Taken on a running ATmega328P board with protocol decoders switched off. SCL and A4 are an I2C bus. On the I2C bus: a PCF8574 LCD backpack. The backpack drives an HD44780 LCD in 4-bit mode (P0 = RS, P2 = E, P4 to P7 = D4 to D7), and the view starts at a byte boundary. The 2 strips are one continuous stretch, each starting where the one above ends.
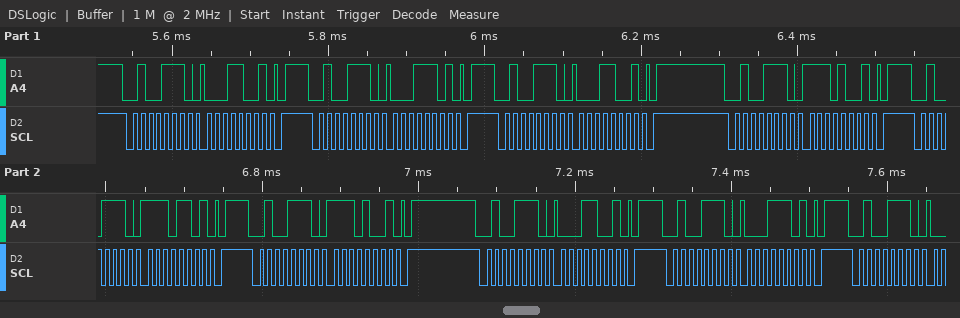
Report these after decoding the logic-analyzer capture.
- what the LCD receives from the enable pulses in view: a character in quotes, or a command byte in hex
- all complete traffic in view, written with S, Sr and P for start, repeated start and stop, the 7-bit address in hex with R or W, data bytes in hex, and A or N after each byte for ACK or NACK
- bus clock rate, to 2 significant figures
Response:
data 0x1E
S 27W A 19 A P S 27W A 1D A P S 27W A 19 A P S 27W A E9 A P S 27W A ED A P S 27W A E9 A P S 27W A 19 A P S 27W A 1D A P S 27W A
100 kHz
